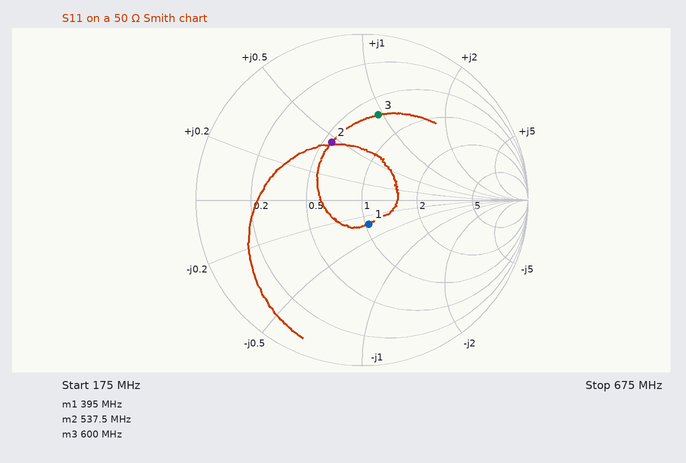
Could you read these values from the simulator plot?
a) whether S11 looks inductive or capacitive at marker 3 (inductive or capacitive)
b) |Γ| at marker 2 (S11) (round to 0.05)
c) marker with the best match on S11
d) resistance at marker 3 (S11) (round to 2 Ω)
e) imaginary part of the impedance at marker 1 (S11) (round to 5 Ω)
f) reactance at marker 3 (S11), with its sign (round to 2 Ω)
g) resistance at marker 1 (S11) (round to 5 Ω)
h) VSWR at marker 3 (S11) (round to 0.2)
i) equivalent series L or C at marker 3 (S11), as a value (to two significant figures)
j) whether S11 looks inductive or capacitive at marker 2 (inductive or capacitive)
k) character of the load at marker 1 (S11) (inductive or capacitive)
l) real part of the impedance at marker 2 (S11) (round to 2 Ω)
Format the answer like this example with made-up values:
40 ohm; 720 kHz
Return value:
inductive; 0.40; marker 1; 34 Ω; -15 Ω; +48 Ω; 50 Ω; 3.2; 13 nH; inductive; capacitive; 28 Ω
